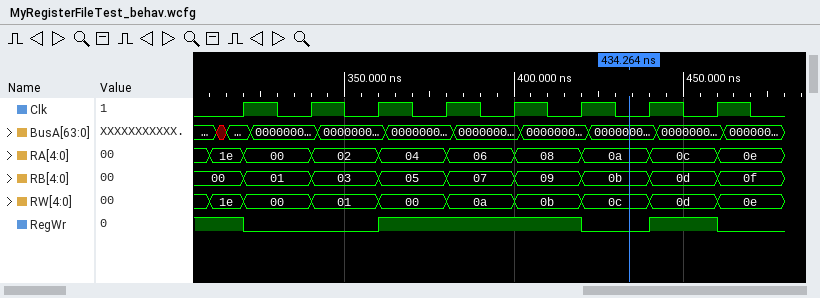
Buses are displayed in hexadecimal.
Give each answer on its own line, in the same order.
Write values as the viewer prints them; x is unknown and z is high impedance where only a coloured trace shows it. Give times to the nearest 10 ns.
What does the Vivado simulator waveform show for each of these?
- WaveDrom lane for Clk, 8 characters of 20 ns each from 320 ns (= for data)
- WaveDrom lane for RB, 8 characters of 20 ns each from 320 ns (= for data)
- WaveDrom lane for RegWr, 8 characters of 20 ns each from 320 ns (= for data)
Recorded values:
{name: 'Clk', wave: 'p.......'}
{name: 'RB', wave: '========', data: '01 03 05 07 09 0b 0d 0f'}
{name: 'RegWr', wave: '0.1..010'}
